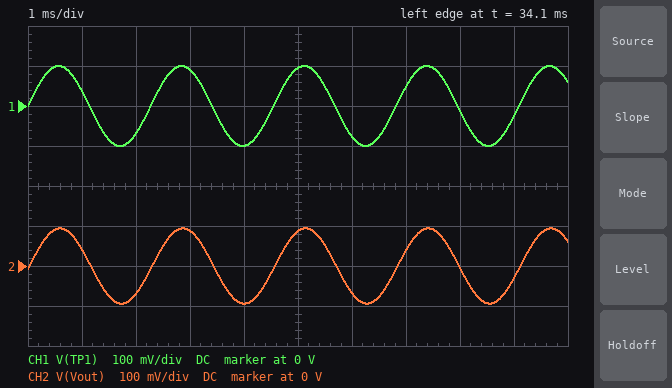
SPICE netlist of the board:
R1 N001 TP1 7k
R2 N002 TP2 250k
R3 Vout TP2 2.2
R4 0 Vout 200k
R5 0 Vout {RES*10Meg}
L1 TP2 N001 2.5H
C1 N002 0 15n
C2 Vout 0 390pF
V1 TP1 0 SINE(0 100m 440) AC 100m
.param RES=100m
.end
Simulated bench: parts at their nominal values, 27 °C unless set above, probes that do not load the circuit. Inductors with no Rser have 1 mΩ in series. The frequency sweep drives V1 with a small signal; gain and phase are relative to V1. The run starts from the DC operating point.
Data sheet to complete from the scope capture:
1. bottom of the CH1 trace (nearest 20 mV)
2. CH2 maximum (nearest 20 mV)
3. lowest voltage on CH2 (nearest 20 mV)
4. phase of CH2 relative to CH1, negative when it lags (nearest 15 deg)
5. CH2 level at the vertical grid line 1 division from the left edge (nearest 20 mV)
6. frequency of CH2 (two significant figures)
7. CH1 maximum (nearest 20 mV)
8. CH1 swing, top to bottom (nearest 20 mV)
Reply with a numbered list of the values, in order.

1. -100 mV
2. 100 mV
3. -100 mV
4. 0 deg
5. 40 mV
6. 440 Hz
7. 100 mV
8. 200 mV
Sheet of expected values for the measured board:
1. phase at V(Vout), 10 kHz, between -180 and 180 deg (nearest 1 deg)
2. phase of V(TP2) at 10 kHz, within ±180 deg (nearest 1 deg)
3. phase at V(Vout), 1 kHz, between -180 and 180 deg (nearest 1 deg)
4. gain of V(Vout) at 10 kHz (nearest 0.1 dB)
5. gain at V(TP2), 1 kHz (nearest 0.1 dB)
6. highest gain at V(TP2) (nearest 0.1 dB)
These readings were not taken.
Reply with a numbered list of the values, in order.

1. -148 deg
2. -148 deg
3. -10 deg
4. -10.3 dB
5. -0.4 dB
6. 1.6 dB
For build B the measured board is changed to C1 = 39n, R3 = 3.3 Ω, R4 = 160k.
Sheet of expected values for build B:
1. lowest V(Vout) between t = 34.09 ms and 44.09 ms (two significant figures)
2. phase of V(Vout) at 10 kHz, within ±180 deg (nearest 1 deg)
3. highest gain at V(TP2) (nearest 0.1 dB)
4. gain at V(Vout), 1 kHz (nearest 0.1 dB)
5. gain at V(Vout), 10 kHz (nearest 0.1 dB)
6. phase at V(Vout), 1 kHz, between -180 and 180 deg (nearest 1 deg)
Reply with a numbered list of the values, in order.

1. -93 mV
2. -145 deg
3. 0.9 dB
4. -0.5 dB
5. -10.6 dB
6. -11 deg
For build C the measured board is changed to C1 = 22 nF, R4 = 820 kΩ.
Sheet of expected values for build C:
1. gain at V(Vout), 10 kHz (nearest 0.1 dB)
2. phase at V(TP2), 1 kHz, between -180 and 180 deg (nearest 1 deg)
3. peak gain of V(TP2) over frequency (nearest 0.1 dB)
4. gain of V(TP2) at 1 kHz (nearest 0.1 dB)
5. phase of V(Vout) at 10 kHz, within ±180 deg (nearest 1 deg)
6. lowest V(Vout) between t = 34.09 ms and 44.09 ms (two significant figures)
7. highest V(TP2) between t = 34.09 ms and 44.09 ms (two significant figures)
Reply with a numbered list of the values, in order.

1. -9.6 dB
2. -7 deg
3. 4.8 dB
4. -0.1 dB
5. -158 deg
6. -97 mV
7. 97 mV
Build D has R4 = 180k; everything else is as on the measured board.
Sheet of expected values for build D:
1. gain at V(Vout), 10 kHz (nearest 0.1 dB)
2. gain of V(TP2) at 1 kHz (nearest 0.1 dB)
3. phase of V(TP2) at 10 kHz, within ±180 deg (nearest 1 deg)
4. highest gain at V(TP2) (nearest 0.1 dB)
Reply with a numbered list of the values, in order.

1. -10.4 dB
2. -0.4 dB
3. -147 deg
4. 1.3 dB
